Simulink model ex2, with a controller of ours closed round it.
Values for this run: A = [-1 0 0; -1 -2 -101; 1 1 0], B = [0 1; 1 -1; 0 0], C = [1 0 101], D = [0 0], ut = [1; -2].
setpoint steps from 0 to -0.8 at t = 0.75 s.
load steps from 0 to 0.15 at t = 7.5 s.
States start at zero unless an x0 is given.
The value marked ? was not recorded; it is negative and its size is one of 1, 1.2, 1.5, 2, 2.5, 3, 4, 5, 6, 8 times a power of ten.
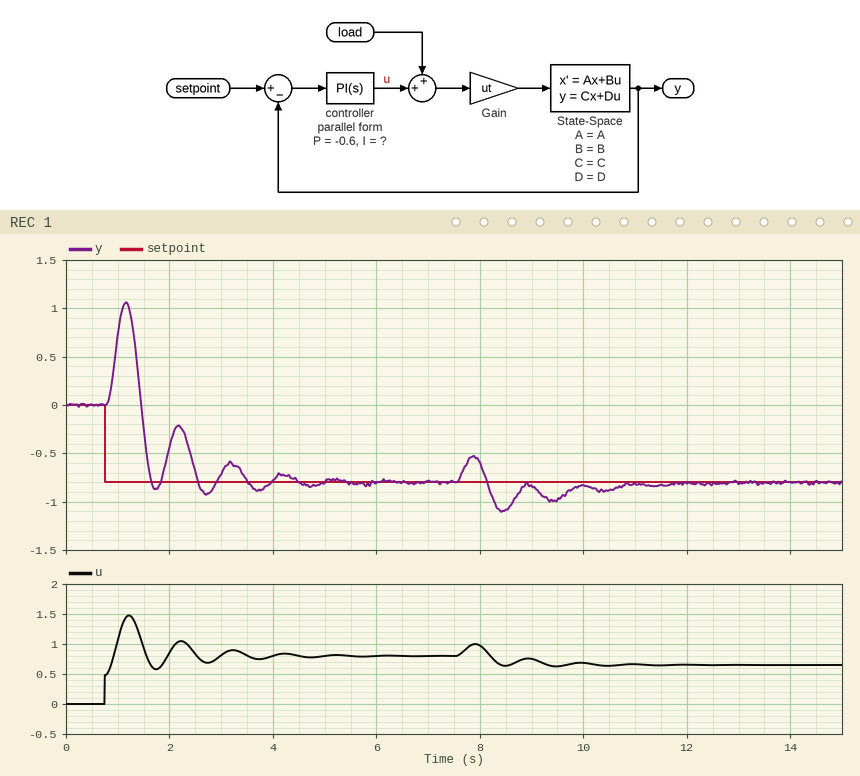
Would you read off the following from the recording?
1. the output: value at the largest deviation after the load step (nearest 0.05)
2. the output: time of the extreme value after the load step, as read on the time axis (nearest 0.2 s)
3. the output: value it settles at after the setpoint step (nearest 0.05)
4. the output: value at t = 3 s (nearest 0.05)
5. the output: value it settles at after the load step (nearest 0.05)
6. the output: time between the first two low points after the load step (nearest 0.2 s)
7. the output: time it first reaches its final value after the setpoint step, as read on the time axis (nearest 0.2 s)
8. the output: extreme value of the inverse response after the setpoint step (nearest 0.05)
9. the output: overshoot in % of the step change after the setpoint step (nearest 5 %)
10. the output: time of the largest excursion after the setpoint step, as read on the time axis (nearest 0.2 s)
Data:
-1.10
8.4 s
-0.80
-0.70
-0.80
1.0 s
1.6 s
1.05
15 %
2.8 s
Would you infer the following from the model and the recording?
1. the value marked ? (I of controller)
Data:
-0.6
